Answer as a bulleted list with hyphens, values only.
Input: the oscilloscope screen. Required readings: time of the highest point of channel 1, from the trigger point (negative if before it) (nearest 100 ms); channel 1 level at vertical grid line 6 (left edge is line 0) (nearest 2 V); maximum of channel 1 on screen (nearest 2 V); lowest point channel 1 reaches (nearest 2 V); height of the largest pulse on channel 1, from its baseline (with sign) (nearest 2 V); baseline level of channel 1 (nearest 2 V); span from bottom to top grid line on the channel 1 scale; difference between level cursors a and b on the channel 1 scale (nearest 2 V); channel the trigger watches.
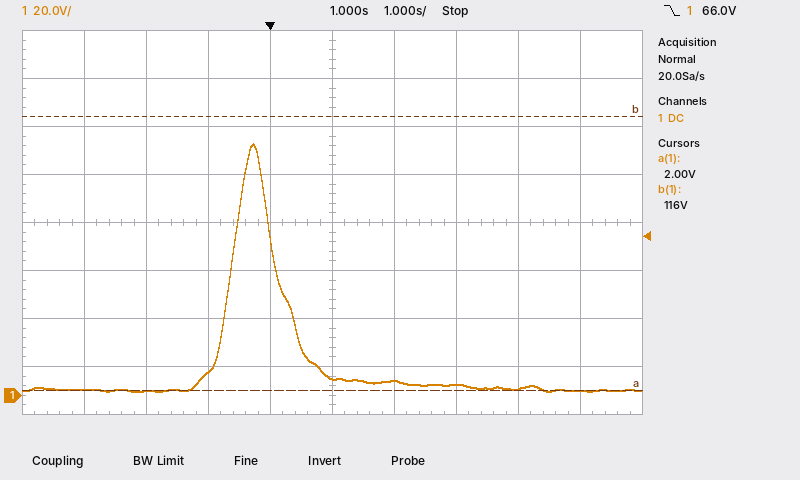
- -300 ms
- 6 V
- 104 V
- 2 V
- +102 V
- 2 V
- 160 V
- 114 V
- channel 1
